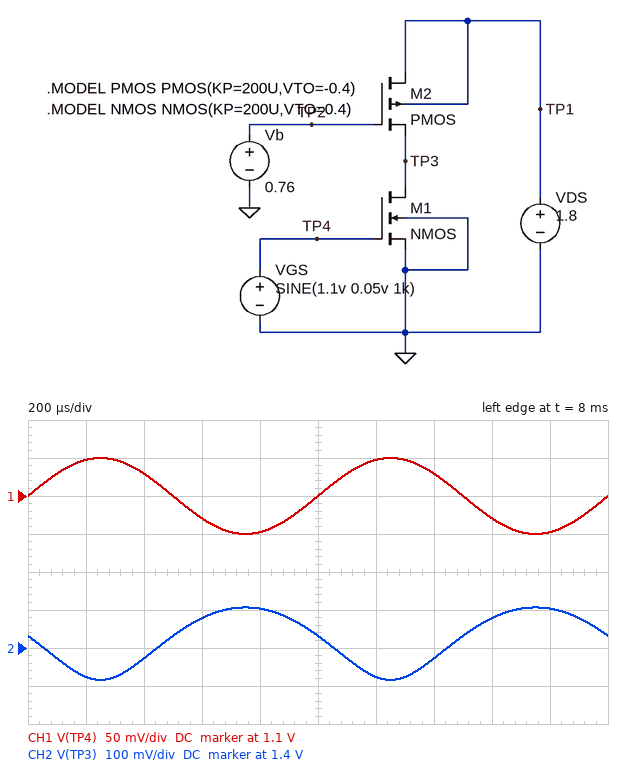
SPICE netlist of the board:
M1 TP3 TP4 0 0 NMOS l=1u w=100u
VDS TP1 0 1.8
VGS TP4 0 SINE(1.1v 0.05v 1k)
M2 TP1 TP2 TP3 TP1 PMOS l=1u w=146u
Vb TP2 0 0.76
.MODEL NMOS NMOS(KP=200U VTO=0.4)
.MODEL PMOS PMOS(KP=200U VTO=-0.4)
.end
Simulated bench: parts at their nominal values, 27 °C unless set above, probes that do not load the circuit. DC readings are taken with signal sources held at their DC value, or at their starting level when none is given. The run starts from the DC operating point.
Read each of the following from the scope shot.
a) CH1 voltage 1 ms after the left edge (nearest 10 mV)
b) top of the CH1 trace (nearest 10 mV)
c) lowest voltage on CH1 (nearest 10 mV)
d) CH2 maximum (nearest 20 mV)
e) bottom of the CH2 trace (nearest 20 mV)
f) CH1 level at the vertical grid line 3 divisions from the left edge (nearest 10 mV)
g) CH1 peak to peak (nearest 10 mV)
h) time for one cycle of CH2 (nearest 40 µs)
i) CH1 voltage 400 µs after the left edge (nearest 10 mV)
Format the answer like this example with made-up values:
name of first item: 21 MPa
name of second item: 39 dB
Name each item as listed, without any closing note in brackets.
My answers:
CH1 voltage 1 ms after the left edge: 1.10 V
top of the CH1 trace: 1.15 V
lowest voltage on CH1: 1.05 V
CH2 maximum: 1.50 V
bottom of the CH2 trace: 1.32 V
CH1 level at the vertical grid line 3 divisions from the left edge: 1.07 V
CH1 peak to peak: 100 mV
time for one cycle of CH2: 1.00 ms
CH1 voltage 400 µs after the left edge: 1.13 V
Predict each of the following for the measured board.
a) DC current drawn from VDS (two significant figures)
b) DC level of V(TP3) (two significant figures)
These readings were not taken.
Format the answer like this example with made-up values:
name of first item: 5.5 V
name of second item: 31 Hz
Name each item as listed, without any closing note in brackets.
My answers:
DC current drawn from VDS: 4.9 mA
DC level of V(TP3): 1.4 V
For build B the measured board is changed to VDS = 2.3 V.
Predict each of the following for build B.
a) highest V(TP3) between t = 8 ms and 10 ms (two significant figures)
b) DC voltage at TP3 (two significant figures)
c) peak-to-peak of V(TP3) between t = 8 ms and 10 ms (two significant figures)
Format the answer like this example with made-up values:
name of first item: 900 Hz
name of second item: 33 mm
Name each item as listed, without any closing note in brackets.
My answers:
highest V(TP3) between t = 8 ms and 10 ms: 2.2 V
DC voltage at TP3: 2.1 V
peak-to-peak of V(TP3) between t = 8 ms and 10 ms: 49 mV
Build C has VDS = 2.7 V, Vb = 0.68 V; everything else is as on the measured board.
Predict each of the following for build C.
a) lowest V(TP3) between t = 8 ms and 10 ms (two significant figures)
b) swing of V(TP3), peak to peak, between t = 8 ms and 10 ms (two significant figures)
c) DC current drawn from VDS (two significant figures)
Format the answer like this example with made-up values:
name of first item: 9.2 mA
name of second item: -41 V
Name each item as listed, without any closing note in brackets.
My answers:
lowest V(TP3) between t = 8 ms and 10 ms: 2.6 V
swing of V(TP3), peak to peak, between t = 8 ms and 10 ms: 32 mV
DC current drawn from VDS: 4.9 mA
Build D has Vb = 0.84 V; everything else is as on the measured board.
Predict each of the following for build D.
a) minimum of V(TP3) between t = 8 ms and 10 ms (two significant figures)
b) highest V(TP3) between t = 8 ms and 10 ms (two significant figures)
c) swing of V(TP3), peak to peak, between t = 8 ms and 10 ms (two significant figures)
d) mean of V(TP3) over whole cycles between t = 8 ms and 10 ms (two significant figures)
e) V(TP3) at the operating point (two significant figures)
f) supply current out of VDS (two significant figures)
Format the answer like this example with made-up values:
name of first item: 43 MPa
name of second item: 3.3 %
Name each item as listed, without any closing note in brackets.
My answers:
minimum of V(TP3) between t = 8 ms and 10 ms: 430 mV
highest V(TP3) between t = 8 ms and 10 ms: 1.4 V
swing of V(TP3), peak to peak, between t = 8 ms and 10 ms: 970 mV
mean of V(TP3) over whole cycles between t = 8 ms and 10 ms: 790 mV
V(TP3) at the operating point: 520 mV
supply current out of VDS: 4.6 mA
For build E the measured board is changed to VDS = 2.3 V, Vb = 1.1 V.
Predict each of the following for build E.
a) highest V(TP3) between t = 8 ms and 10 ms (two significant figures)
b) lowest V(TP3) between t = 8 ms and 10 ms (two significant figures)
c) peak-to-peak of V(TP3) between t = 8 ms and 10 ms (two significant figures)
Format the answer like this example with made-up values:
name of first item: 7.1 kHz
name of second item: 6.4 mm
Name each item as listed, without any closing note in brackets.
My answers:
highest V(TP3) between t = 8 ms and 10 ms: 2.1 V
lowest V(TP3) between t = 8 ms and 10 ms: 2.0 V
peak-to-peak of V(TP3) between t = 8 ms and 10 ms: 87 mV
